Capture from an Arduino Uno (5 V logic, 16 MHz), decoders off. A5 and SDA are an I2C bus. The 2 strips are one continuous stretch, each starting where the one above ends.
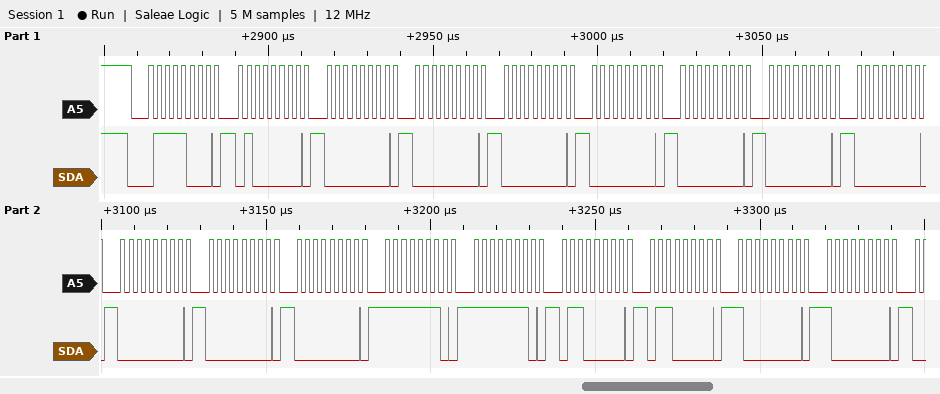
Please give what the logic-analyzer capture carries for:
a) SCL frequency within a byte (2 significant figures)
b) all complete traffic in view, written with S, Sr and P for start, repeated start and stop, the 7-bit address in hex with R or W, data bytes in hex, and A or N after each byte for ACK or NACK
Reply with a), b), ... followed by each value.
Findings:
a) 400 kHz
b) S 3CW A 40 A 00 A 00 A 00 A 00 A 00 A 00 A 00 A 00 A 00 A 00 A FE A FE A 60 A 60 A 80 A 80 A
